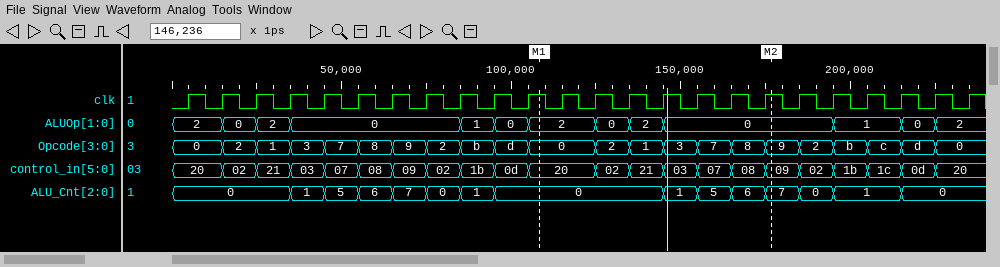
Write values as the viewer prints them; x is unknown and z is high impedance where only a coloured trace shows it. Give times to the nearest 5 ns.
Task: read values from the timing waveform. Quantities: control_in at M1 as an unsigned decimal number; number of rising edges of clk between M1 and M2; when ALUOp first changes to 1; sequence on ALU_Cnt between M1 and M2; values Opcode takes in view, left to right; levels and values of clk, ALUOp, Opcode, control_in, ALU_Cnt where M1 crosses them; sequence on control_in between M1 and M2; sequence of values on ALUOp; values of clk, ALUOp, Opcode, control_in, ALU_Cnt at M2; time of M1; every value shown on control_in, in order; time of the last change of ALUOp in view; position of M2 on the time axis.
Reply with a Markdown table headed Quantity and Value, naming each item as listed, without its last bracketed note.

| Quantity | Value |
|---|---|
| control_in at M1 as an unsigned decimal number | 32 |
| number of rising edges of clk between M1 and M2 | 7 |
| when ALUOp first changes to 1 | 85 ns |
| sequence on ALU_Cnt between M1 and M2 | 0, 1, 5, 6, 7 |
| values Opcode takes in view, left to right | 0, 2, 1, 3, 7, 8, 9, 2, b, d, 0, 2, 1, 3, 7, 8, 9, 2, b, c, d, 0 |
| levels and values of clk, ALUOp, Opcode, control_in, ALU_Cnt where M1 crosses them | clk=1, ALUOp=2, Opcode=0, control_in=20, ALU_Cnt=0 |
| sequence on control_in between M1 and M2 | 20, 02, 21, 03, 07, 08, 09 |
| sequence of values on ALUOp | 2, 0, 2, 0, 1, 0, 2, 0, 2, 0, 1, 0, 2 |
| values of clk, ALUOp, Opcode, control_in, ALU_Cnt at M2 | clk=1, ALUOp=0, Opcode=9, control_in=09, ALU_Cnt=7 |
| time of M1 | 110 ns |
| every value shown on control_in, in order | 20, 02, 21, 03, 07, 08, 09, 02, 1b, 0d, 20, 02, 21, 03, 07, 08, 09, 02, 1b, 1c, 0d, 20 |
| time of the last change of ALUOp in view | 225 ns |
| position of M2 on the time axis | 175 ns |
